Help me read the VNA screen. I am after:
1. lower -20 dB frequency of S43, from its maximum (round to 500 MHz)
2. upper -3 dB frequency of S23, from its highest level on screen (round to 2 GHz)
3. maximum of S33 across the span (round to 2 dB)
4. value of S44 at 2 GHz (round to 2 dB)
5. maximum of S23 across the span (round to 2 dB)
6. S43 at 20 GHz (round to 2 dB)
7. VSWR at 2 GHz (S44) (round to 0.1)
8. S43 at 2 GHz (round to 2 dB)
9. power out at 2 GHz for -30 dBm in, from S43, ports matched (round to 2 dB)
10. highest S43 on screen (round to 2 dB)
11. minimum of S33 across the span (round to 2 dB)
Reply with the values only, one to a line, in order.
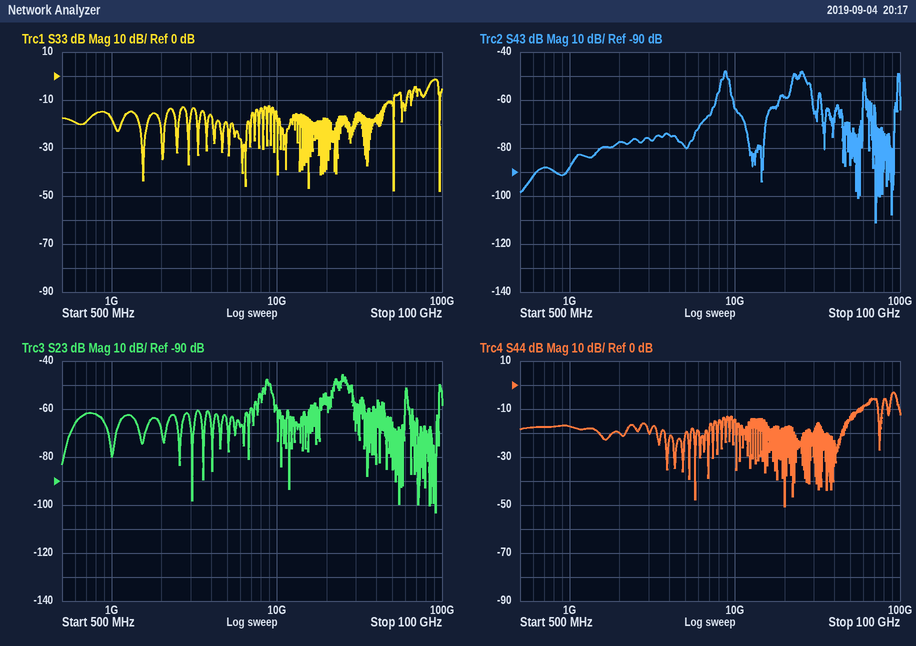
6.5 GHz
26 GHz
-2 dB
-20 dB
-46 dB
-58 dB
1.2
-78 dB
-108 dBm
-48 dB
-48 dB
